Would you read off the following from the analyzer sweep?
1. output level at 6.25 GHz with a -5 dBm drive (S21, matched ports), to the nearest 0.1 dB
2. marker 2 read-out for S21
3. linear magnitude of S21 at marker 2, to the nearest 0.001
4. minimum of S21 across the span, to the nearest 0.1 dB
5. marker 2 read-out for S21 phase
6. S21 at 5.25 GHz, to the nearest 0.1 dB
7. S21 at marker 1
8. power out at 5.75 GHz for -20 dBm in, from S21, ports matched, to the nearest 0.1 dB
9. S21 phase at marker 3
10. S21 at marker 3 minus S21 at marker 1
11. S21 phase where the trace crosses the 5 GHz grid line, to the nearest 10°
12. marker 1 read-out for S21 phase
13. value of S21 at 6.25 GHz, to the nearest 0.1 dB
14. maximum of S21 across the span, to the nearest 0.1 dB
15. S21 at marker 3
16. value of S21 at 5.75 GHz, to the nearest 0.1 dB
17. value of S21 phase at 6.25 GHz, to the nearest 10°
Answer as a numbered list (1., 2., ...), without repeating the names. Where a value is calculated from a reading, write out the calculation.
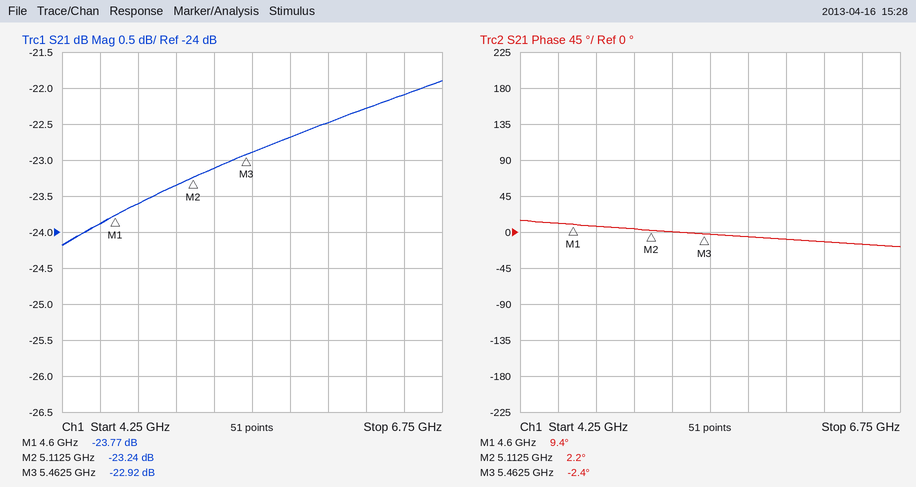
1. -5 dBm + (-22.3 dB) = -27.3 dBm
2. -23.24 dB
3. 10^(-23.24/20) ≈ 0.069
4. -24.2 dB
5. 2.2°
6. -23.1 dB
7. -23.77 dB
8. -20 dBm + (-22.7 dB) = -42.7 dBm
9. -2.4°
10. -22.92 − (-23.77) = 0.85 dB
11. 0°
12. 9.4°
13. -22.3 dB
14. -21.9 dB
15. -22.92 dB
16. -22.7 dB
17. -10°
